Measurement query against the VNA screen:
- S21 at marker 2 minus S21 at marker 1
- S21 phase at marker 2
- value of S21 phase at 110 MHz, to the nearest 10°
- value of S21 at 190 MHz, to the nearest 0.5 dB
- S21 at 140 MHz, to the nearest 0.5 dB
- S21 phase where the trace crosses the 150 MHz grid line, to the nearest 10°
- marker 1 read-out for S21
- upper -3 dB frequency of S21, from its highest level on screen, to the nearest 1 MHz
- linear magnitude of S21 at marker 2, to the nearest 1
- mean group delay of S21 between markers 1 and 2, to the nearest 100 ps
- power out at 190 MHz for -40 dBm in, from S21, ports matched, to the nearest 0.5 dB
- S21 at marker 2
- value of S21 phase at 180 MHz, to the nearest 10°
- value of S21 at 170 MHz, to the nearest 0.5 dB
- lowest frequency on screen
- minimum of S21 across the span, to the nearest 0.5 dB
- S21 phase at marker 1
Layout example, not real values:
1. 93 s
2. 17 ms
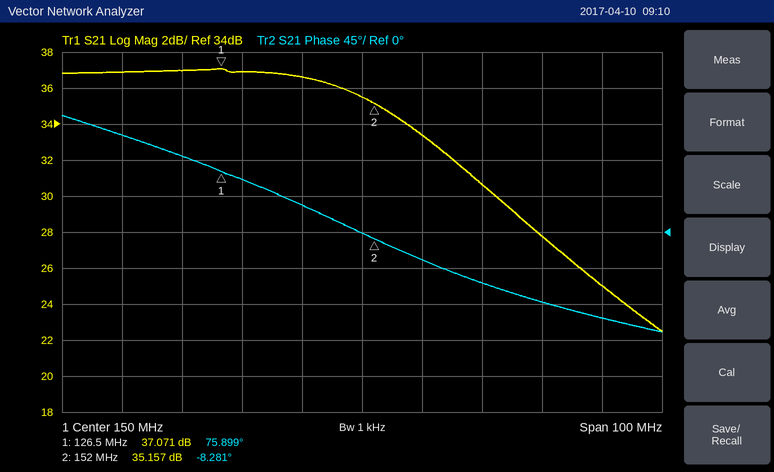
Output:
1. -1.914 dB
2. -8.281°
3. 120°
4. 25.0 dB
5. 36.5 dB
6. 0°
7. 37.071 dB
8. 157 MHz
9. 57
10. 9.2 ns
11. -15.0 dBm
12. 35.157 dB
13. -90°
14. 30.5 dB
15. 100 MHz
16. 22.5 dB
17. 75.899°
